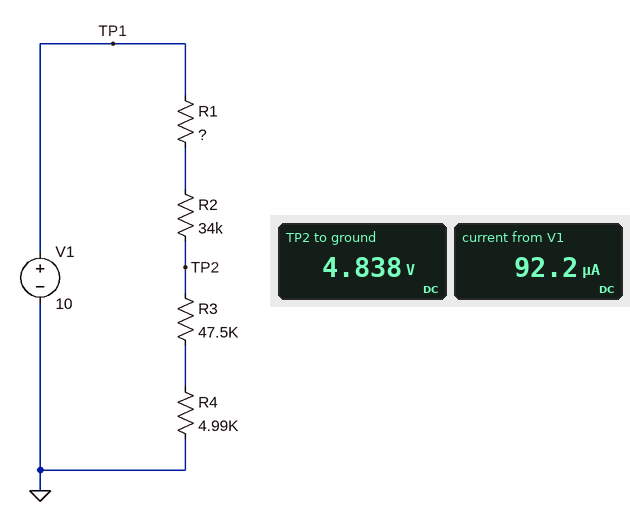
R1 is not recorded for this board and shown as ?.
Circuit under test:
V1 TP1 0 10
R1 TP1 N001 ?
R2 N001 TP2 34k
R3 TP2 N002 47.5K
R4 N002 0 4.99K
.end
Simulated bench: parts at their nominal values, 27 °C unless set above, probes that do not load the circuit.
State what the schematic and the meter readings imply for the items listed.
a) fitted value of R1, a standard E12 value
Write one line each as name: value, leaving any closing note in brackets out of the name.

fitted value of R1, a standard E12 value: 22 kΩ
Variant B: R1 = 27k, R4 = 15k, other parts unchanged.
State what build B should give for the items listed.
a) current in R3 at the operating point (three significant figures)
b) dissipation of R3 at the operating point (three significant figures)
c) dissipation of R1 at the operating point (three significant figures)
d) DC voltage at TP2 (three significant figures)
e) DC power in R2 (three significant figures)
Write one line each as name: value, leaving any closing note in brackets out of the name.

current in R3 at the operating point: 81.0 µA
dissipation of R3 at the operating point: 311 µW
dissipation of R1 at the operating point: 177 µW
DC voltage at TP2: 5.06 V
DC power in R2: 223 µW
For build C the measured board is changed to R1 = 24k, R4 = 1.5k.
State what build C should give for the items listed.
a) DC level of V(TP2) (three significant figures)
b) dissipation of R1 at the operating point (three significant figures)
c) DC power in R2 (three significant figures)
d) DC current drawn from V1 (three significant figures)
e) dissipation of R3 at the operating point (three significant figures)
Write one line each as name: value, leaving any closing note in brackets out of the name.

DC level of V(TP2): 4.58 V
dissipation of R1 at the operating point: 210 µW
DC power in R2: 297 µW
DC current drawn from V1: 93.5 µA
dissipation of R3 at the operating point: 415 µW
